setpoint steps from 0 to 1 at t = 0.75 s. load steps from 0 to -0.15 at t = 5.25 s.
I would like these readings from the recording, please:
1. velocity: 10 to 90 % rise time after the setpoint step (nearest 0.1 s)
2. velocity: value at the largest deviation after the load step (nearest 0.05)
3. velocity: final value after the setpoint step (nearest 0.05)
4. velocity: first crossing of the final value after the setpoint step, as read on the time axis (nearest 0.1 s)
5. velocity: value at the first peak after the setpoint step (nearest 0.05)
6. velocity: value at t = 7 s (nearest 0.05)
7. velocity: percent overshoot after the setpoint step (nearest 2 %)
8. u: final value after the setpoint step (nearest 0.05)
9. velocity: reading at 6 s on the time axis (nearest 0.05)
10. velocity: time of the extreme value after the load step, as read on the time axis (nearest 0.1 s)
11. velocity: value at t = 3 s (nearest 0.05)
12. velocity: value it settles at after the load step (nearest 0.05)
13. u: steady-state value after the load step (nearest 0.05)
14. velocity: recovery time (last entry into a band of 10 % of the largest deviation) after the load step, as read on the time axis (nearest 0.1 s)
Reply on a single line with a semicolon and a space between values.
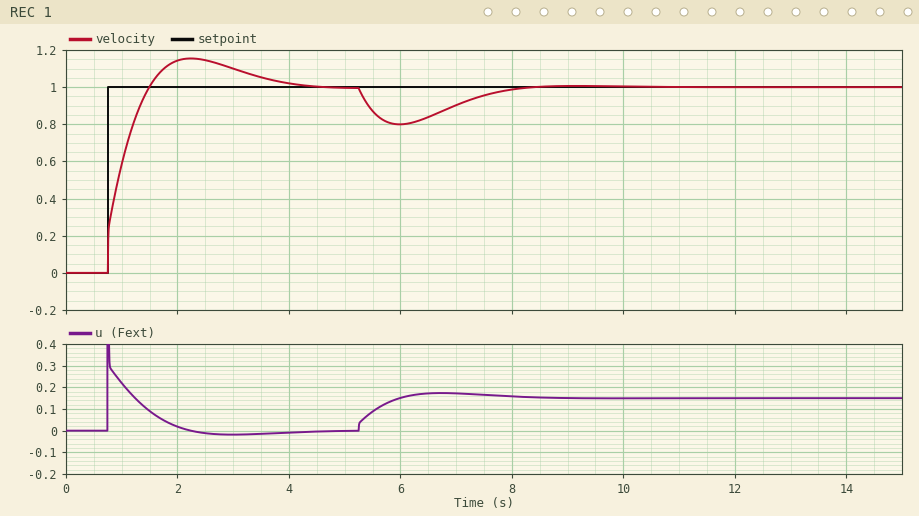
0.6 s; 0.80; 1.00; 1.5 s; 1.15; 0.90; 16 %; 0.00; 0.80; 6.0 s; 1.10; 1.00; 0.15; 7.9 s
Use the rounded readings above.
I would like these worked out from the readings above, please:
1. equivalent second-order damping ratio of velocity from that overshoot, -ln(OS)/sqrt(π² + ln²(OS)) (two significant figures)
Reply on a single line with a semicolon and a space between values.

0.50
